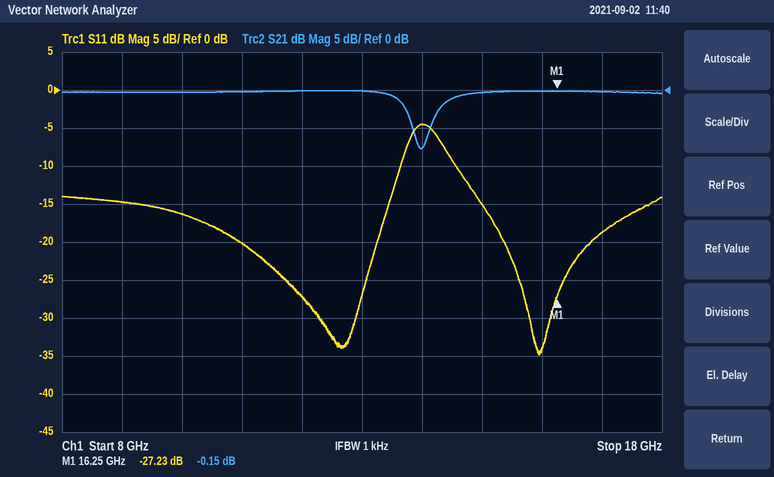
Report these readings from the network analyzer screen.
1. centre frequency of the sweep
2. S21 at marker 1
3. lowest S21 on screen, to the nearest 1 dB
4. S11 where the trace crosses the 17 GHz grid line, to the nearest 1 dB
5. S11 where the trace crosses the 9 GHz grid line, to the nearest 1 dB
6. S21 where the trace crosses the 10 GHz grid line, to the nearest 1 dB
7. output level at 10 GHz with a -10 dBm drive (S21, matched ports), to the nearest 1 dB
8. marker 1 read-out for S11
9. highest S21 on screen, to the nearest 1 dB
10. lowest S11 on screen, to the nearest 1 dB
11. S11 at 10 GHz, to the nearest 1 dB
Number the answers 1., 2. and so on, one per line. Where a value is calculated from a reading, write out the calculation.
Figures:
1. 13 GHz
2. -0.15 dB
3. -8 dB
4. -19 dB
5. -15 dB
6. 0 dB
7. -10 dBm + (0 dB) = -10 dBm
8. -27.23 dB
9. 0 dB
10. -35 dB
11. -16 dB
